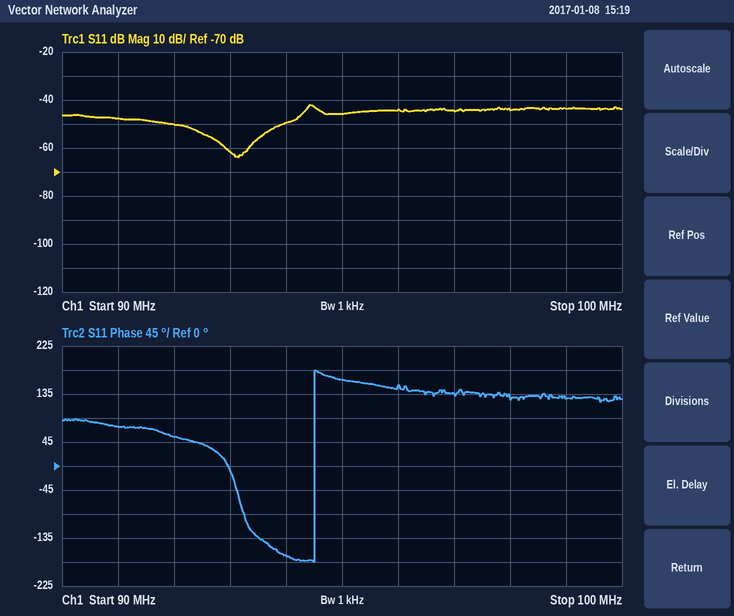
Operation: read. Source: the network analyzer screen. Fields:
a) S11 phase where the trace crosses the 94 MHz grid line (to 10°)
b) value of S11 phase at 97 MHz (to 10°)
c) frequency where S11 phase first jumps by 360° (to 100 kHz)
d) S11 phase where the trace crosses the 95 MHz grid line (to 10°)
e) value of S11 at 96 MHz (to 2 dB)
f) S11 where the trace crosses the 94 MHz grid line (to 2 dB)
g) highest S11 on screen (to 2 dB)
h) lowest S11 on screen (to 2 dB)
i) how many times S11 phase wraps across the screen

-170°
140°
94.5 MHz
160°
-44 dB
-50 dB
-42 dB
-64 dB
1
